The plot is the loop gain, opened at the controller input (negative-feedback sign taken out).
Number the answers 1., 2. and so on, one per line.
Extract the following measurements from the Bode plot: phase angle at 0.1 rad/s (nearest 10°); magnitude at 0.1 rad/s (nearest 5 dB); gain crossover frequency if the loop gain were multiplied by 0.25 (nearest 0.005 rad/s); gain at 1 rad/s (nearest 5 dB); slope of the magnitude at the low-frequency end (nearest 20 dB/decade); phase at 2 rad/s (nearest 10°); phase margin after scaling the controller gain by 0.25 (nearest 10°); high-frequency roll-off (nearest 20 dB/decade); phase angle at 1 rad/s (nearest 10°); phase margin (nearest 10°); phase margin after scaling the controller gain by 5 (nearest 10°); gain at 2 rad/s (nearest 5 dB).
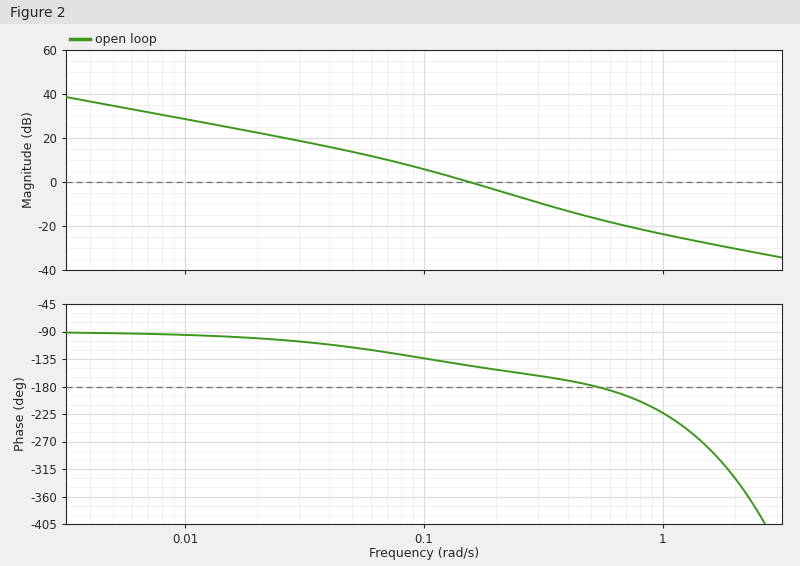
1. -130°
2. 5 dB
3. 0.060 rad/s
4. -25 dB
5. -20 dB/decade
6. -330°
7. 60°
8. -20 dB/decade
9. -220°
10. 30°
11. 10°
12. -30 dB
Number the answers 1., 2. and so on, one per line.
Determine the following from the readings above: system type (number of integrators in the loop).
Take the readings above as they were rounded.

1. 1
